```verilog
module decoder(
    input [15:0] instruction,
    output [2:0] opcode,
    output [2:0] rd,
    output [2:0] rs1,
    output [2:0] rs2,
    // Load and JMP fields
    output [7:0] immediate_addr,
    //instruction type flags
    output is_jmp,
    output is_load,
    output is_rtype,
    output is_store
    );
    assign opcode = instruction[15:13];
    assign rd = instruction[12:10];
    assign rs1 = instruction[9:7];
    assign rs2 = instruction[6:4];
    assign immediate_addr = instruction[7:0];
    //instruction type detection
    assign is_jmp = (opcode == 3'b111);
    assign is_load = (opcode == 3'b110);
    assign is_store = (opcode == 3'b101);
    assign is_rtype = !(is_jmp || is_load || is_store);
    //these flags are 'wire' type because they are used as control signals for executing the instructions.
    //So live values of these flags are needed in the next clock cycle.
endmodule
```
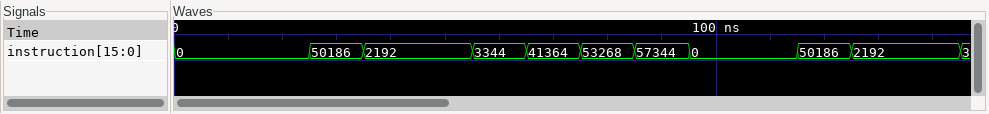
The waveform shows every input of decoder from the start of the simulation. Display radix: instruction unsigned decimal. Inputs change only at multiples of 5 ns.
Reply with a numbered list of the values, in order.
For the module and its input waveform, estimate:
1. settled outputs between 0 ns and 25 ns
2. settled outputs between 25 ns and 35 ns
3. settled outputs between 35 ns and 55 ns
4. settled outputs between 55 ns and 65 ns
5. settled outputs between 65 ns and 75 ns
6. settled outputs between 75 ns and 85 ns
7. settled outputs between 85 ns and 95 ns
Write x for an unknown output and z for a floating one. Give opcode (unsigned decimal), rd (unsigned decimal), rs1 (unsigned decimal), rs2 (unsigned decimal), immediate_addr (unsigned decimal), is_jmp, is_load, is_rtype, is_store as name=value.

1. opcode=0, rd=0, rs1=0, rs2=0, immediate_addr=0, is_jmp=0, is_load=0, is_rtype=1, is_store=0
2. opcode=6, rd=1, rs1=0, rs2=0, immediate_addr=10, is_jmp=0, is_load=1, is_rtype=0, is_store=0
3. opcode=0, rd=2, rs1=1, rs2=1, immediate_addr=144, is_jmp=0, is_load=0, is_rtype=1, is_store=0
4. opcode=0, rd=3, rs1=2, rs2=1, immediate_addr=16, is_jmp=0, is_load=0, is_rtype=1, is_store=0
5. opcode=5, rd=0, rs1=3, rs2=1, immediate_addr=148, is_jmp=0, is_load=0, is_rtype=0, is_store=1
6. opcode=6, rd=4, rs1=0, rs2=1, immediate_addr=20, is_jmp=0, is_load=1, is_rtype=0, is_store=0
7. opcode=7, rd=0, rs1=0, rs2=0, immediate_addr=0, is_jmp=1, is_load=0, is_rtype=0, is_store=0
